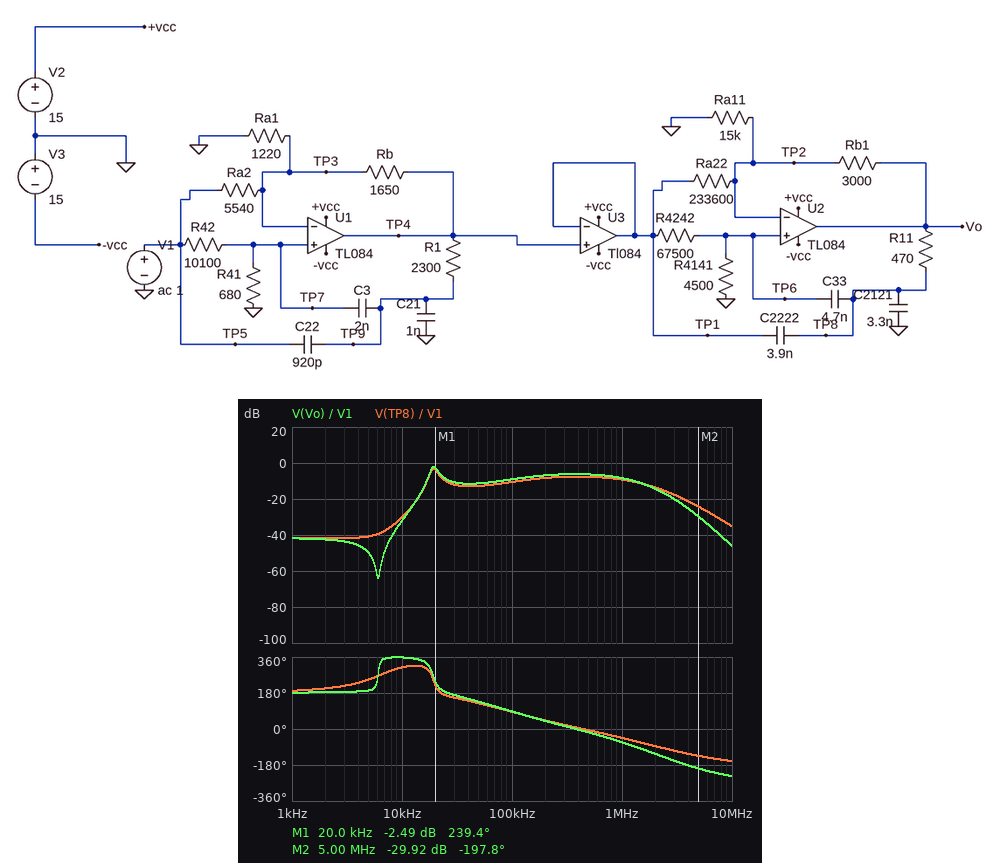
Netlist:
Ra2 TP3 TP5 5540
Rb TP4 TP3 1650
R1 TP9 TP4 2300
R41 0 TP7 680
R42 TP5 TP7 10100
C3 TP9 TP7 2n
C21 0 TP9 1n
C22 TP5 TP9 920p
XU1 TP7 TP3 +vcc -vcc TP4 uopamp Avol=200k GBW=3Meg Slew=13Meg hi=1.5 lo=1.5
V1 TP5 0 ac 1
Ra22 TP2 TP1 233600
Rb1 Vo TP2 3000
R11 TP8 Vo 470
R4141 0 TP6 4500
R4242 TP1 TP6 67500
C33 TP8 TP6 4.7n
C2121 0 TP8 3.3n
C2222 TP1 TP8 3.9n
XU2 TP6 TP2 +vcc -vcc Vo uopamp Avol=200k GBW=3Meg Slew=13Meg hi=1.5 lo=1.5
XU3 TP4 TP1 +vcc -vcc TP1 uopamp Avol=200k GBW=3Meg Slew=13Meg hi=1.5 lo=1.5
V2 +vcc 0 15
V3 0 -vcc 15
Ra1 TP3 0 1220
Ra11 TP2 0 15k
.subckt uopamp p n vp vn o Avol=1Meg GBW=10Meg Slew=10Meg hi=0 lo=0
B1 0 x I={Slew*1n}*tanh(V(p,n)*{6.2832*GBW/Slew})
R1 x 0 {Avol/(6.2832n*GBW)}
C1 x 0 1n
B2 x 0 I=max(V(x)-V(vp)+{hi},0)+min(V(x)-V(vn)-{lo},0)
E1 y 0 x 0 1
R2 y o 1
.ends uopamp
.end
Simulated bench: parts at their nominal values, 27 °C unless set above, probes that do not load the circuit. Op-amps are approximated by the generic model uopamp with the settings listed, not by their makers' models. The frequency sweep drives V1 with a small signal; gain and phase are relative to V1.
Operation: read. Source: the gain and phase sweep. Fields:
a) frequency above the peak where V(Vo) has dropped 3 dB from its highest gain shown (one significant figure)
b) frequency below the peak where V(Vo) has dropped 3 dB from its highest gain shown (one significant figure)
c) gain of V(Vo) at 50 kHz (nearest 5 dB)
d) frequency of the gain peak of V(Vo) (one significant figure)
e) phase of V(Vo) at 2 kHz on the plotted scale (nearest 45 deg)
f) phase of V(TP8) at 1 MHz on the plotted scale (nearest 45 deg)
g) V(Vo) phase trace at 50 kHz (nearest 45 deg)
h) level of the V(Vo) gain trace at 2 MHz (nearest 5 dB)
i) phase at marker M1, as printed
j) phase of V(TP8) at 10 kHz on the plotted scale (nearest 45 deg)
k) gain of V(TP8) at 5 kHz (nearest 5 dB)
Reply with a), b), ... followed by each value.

a) 20 kHz
b) 20 kHz
c) -10 dB
d) 20 kHz
e) 180 deg
f) -45 deg
g) 135 deg
h) -15 dB
i) 239.4 deg
j) 315 deg
k) -40 dB
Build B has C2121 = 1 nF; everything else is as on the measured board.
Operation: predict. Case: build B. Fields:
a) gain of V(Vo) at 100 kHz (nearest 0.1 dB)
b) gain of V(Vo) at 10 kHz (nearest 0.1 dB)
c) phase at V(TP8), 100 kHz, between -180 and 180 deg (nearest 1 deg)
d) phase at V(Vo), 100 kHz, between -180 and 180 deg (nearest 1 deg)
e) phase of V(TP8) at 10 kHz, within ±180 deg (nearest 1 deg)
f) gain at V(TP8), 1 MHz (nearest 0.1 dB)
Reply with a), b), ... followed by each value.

a) -5.6 dB
b) -32.9 dB
c) 85 deg
d) 87 deg
e) -46 deg
f) -6.0 dB
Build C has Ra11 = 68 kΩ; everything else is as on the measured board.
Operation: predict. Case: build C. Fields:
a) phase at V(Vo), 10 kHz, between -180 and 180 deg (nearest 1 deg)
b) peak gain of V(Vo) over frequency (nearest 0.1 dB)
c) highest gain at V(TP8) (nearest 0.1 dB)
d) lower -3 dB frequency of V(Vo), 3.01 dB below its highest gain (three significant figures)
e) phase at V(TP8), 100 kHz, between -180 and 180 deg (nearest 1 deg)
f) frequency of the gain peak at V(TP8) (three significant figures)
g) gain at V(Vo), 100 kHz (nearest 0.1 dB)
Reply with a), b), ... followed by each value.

a) -15 deg
b) -7.3 dB
c) -7.5 dB
d) 98.4 kHz
e) 90 deg
f) 396 kHz
g) -10.3 dB
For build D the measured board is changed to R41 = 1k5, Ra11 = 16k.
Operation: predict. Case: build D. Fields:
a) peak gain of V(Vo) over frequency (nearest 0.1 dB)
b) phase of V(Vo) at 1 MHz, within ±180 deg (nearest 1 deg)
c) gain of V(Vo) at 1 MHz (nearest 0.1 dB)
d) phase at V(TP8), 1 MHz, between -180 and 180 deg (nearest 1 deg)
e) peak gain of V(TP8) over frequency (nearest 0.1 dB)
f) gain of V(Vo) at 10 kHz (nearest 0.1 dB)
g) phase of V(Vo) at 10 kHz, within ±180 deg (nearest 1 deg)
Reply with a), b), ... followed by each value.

a) -4.9 dB
b) -75 deg
c) -8.3 dB
d) -54 deg
e) -6.3 dB
f) -49.3 dB
g) 62 deg
